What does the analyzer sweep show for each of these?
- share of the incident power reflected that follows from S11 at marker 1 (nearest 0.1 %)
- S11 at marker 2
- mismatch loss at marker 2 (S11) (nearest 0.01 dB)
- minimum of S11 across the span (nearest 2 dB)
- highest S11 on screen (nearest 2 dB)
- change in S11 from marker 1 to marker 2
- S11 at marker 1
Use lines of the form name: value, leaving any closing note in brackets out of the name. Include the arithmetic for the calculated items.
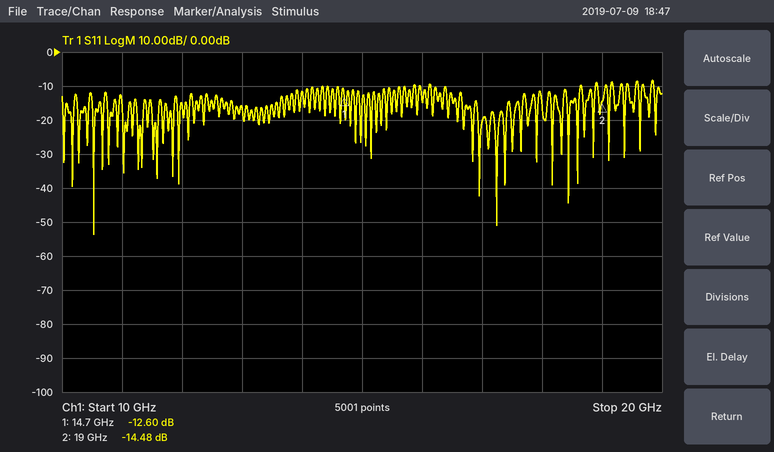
share of the incident power reflected that follows from S11 at marker 1: 10^(-12.6/10) ≈ 5.5 %
S11 at marker 2: -14.48 dB
mismatch loss at marker 2 (S11): −10 log10(1 − 10^(-14.48/10)) ≈ 0.16 dB
minimum of S11 across the span: -54 dB
highest S11 on screen: -8 dB
change in S11 from marker 1 to marker 2: -14.48 − (-12.6) = -1.88 dB
S11 at marker 1: -12.60 dB
